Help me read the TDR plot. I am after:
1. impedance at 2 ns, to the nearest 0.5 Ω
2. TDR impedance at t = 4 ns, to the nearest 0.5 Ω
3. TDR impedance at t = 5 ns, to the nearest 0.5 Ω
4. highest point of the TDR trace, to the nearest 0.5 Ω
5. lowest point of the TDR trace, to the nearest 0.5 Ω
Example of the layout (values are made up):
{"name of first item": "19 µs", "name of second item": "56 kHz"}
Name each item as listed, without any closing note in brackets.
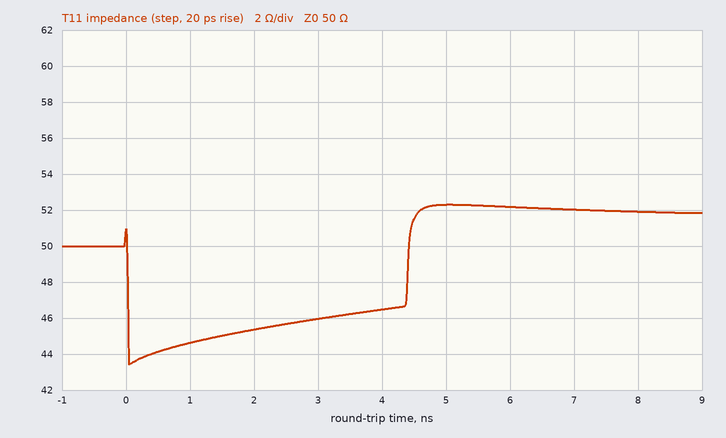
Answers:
{"impedance at 2 ns, to the nearest 0.5 Ω": "45.5 Ω", "TDR impedance at t = 4 ns, to the nearest 0.5 Ω": "46.5 Ω", "TDR impedance at t = 5 ns, to the nearest 0.5 Ω": "52.5 Ω", "highest point of the TDR trace, to the nearest 0.5 Ω": "52.5 Ω", "lowest point of the TDR trace, to the nearest 0.5 Ω": "43.5 Ω"}
